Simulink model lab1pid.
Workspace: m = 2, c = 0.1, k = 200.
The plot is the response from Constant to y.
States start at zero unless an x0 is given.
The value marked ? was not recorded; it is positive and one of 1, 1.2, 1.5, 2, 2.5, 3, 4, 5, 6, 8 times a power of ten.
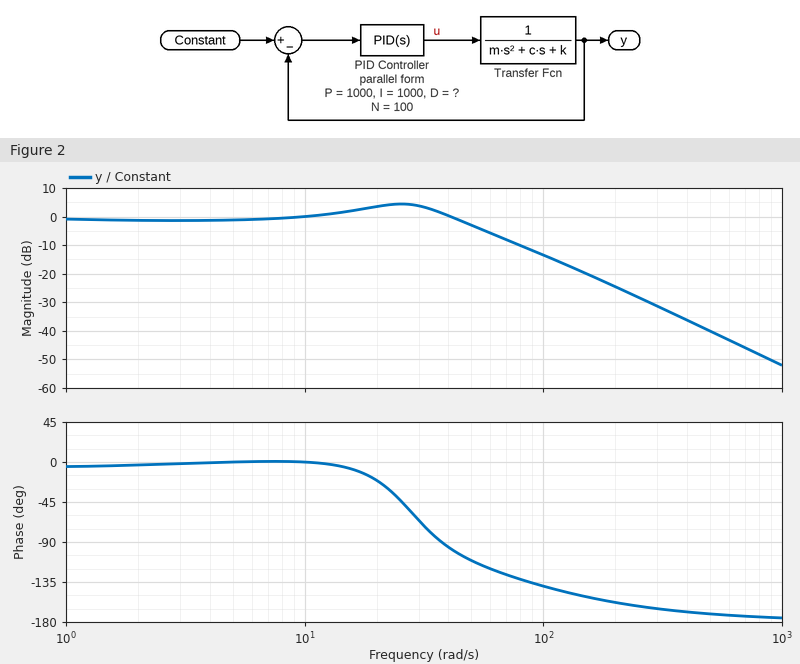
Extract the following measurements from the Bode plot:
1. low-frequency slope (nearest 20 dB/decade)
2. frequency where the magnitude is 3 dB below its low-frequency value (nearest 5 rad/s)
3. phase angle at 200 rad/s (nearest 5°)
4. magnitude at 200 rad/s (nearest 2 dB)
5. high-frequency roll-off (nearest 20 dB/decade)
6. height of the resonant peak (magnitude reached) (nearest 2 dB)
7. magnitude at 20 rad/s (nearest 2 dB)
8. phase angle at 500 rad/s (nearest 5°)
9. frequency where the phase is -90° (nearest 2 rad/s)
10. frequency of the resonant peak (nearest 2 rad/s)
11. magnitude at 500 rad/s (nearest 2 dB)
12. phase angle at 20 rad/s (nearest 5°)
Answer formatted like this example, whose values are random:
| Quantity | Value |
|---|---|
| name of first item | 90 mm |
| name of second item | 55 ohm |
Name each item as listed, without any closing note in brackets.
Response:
| Quantity | Value |
|---|---|
| low-frequency slope | 0 dB/decade |
| frequency where the magnitude is 3 dB below its low-frequency value | 55 rad/s |
| phase angle at 200 rad/s | -160° |
| magnitude at 200 rad/s | -24 dB |
| high-frequency roll-off | -40 dB/decade |
| height of the resonant peak (magnitude reached) | 4 dB |
| magnitude at 20 rad/s | 4 dB |
| phase angle at 500 rad/s | -170° |
| frequency where the phase is -90° | 38 rad/s |
| frequency of the resonant peak | 26 rad/s |
| magnitude at 500 rad/s | -40 dB |
| phase angle at 20 rad/s | -20° |
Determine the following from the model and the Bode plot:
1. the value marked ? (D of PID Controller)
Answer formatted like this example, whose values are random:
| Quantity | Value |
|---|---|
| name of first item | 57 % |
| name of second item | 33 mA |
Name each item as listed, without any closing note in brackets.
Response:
| Quantity | Value |
|---|---|
| the value marked ? | 40 |
